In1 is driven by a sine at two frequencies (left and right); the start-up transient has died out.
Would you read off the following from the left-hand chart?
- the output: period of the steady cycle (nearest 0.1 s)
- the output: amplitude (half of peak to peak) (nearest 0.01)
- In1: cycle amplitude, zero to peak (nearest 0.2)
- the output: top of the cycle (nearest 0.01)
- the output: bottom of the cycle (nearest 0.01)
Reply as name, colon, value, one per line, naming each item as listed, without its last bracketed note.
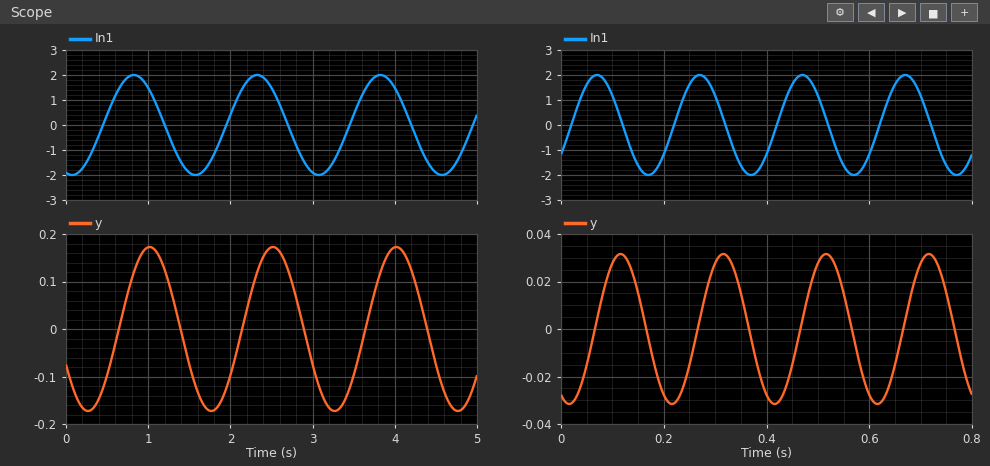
the output: period of the steady cycle: 1.5 s
the output: amplitude (half of peak to peak): 0.17
In1: cycle amplitude, zero to peak: 2.0
the output: top of the cycle: 0.17
the output: bottom of the cycle: -0.17
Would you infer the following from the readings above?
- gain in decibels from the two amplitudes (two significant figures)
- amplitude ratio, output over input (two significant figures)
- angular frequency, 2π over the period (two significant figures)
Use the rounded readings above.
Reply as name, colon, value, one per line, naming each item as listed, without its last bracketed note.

gain in decibels from the two amplitudes: -21 dB
amplitude ratio, output over input: 0.085
angular frequency, 2π over the period: 4.2 rad/s
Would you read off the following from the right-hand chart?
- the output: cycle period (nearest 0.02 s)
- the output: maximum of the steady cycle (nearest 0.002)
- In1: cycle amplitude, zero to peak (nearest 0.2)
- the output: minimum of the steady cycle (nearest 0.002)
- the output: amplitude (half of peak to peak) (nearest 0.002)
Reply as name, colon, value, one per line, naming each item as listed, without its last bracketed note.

the output: cycle period: 0.20 s
the output: maximum of the steady cycle: 0.032
In1: cycle amplitude, zero to peak: 2.0
the output: minimum of the steady cycle: -0.032
the output: amplitude (half of peak to peak): 0.032
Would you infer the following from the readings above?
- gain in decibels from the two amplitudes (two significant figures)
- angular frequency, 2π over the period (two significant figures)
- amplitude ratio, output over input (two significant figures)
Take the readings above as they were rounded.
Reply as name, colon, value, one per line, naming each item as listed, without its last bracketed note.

gain in decibels from the two amplitudes: -36 dB
angular frequency, 2π over the period: 31 rad/s
amplitude ratio, output over input: 0.016
